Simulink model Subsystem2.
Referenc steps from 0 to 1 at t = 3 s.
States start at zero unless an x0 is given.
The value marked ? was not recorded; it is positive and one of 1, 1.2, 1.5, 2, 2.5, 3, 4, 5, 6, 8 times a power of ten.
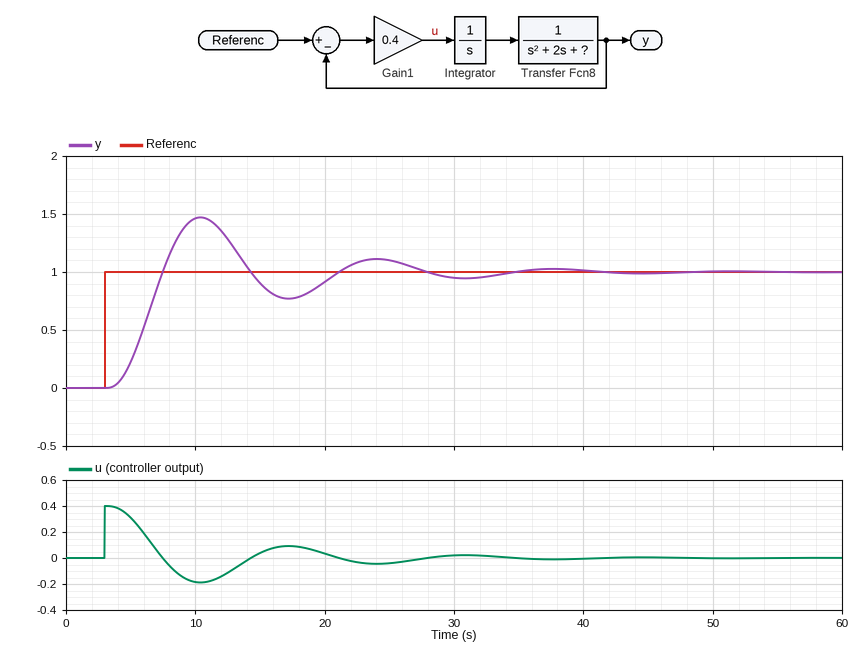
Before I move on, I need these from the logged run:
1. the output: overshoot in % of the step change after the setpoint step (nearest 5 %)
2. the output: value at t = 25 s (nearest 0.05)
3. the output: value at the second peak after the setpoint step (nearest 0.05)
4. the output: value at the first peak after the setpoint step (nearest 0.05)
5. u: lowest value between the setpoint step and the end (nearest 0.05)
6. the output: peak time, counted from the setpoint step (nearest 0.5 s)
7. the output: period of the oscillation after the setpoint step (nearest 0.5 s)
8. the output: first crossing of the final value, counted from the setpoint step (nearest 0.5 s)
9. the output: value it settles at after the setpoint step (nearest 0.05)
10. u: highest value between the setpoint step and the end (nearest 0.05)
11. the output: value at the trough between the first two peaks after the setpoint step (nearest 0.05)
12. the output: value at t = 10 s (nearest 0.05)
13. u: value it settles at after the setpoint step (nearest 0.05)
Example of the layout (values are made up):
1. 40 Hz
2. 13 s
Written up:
1. 45 %
2. 1.10
3. 1.10
4. 1.45
5. -0.20
6. 7.5 s
7. 13.5 s
8. 4.5 s
9. 1.00
10. 0.40
11. 0.75
12. 1.45
13. 0.00
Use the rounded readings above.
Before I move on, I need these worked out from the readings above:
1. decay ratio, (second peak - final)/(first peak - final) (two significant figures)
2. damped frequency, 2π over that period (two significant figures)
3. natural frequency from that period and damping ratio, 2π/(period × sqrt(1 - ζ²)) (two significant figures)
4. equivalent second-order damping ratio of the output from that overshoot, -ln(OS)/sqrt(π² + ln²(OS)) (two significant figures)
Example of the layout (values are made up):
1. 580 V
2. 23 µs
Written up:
1. 0.22
2. 0.47 rad/s
3. 0.48 rad/s
4. 0.25
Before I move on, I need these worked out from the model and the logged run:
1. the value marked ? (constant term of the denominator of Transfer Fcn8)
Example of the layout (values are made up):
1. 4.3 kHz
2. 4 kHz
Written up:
1. 0.6
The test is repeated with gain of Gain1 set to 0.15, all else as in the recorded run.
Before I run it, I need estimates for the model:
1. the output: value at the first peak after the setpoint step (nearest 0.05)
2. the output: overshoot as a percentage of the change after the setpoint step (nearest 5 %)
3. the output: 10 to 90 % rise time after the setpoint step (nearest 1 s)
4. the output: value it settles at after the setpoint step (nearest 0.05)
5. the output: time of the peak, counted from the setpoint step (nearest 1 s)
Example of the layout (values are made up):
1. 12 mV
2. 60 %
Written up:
1. 1.15
2. 15 %
3. 6 s
4. 1.00
5. 13 s
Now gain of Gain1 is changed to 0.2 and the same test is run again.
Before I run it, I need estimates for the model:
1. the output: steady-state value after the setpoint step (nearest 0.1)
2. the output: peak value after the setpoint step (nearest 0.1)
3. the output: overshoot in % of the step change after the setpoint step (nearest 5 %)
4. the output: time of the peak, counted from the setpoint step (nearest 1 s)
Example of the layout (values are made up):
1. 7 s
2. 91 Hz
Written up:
1. 1.0
2. 1.2
3. 25 %
4. 11 s
